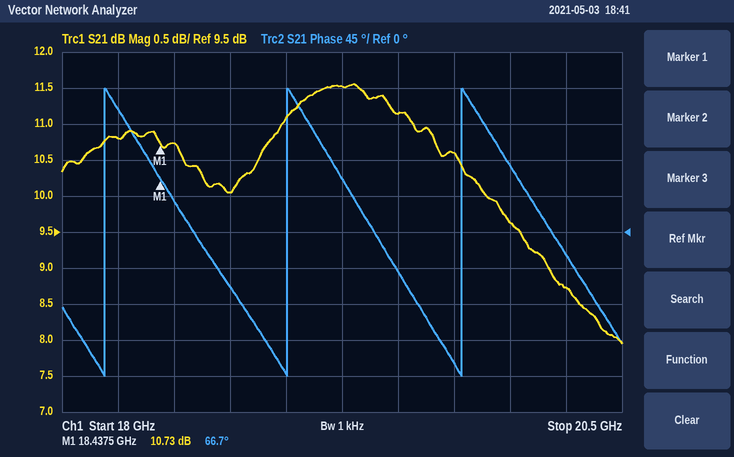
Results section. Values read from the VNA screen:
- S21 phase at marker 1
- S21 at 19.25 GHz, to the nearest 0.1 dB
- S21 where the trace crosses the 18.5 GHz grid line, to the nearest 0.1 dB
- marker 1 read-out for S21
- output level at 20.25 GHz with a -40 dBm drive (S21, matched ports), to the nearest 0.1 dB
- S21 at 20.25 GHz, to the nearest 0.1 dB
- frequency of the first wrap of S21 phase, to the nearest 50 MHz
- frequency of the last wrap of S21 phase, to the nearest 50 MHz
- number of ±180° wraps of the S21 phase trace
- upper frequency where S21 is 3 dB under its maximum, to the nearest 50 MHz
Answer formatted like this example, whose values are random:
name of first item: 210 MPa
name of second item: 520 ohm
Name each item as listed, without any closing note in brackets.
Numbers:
S21 phase at marker 1: 66.7°
S21 at 19.25 GHz, to the nearest 0.1 dB: 11.5 dB
S21 where the trace crosses the 18.5 GHz grid line, to the nearest 0.1 dB: 10.7 dB
marker 1 read-out for S21: 10.73 dB
output level at 20.25 GHz with a -40 dBm drive (S21, matched ports), to the nearest 0.1 dB: -31.3 dBm
S21 at 20.25 GHz, to the nearest 0.1 dB: 8.7 dB
frequency of the first wrap of S21 phase, to the nearest 50 MHz: 18.20 GHz
frequency of the last wrap of S21 phase, to the nearest 50 MHz: 19.80 GHz
number of ±180° wraps of the S21 phase trace: 3
upper frequency where S21 is 3 dB under its maximum, to the nearest 50 MHz: 20.30 GHz
